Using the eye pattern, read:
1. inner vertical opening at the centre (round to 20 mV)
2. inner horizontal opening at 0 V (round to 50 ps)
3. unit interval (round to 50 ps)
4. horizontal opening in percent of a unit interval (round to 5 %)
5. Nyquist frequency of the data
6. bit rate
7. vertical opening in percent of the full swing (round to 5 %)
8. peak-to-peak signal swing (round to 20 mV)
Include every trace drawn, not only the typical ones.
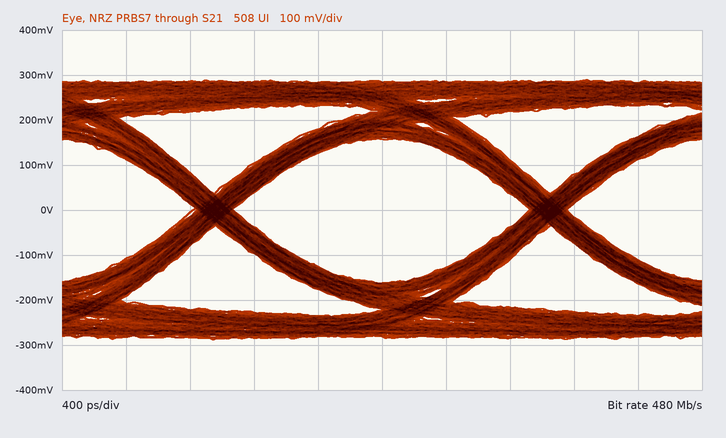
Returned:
320 mV
1.85 ns
2.10 ns
90 %
240 MHz
480 Mb/s
55 %
580 mV
